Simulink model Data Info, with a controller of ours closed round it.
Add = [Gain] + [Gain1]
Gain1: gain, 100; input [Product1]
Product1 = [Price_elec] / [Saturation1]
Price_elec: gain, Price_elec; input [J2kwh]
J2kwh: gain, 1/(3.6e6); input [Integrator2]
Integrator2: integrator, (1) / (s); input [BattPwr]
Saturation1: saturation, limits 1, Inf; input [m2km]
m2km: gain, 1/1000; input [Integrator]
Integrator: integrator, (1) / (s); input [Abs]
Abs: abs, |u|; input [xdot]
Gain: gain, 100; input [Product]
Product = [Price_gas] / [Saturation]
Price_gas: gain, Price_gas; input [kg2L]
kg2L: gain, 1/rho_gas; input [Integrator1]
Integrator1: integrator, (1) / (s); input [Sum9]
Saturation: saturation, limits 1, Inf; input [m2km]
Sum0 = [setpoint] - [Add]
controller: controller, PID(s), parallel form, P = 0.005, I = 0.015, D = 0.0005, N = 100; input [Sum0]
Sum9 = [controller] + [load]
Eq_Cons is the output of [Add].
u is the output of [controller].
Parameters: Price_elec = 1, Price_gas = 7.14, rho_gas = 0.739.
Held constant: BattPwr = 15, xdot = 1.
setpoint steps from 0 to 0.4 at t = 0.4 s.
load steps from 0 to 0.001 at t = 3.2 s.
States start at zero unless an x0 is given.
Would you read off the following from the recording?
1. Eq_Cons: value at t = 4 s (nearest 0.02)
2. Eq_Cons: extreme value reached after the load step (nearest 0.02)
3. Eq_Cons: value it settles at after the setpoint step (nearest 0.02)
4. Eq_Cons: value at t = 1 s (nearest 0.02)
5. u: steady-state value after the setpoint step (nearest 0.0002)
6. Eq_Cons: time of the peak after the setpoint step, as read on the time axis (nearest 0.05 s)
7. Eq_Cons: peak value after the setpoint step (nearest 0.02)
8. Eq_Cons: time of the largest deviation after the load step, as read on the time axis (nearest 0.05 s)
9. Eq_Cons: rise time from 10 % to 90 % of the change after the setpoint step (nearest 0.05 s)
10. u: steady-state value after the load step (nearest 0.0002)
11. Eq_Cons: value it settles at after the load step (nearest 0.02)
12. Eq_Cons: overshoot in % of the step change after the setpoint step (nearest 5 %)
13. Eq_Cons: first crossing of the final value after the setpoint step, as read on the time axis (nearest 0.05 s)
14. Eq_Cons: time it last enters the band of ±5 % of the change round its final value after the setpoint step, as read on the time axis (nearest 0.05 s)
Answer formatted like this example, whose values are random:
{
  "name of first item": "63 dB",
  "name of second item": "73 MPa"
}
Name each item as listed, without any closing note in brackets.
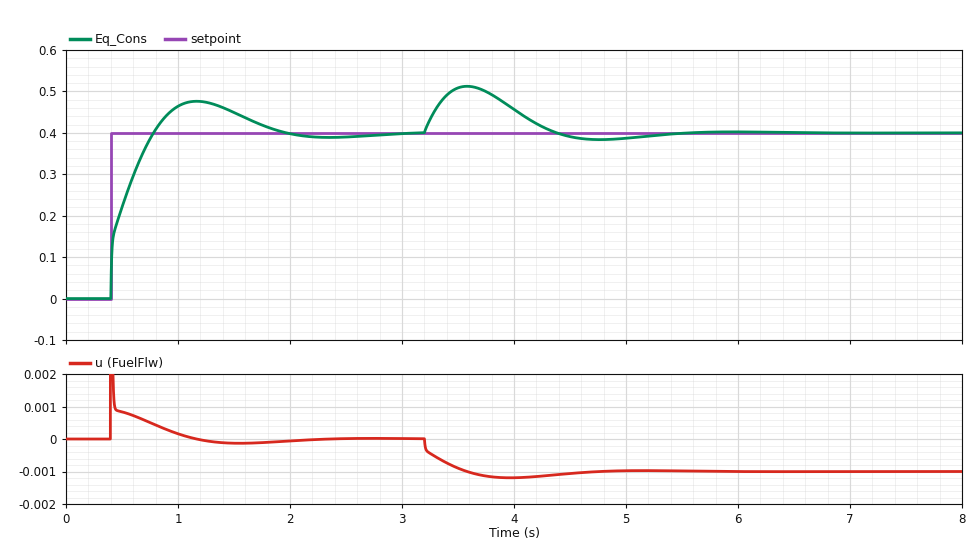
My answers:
{
  "Eq_Cons: value at t = 4 s": "0.46",
  "Eq_Cons: extreme value reached after the load step": "0.52",
  "Eq_Cons: value it settles at after the setpoint step": "0.40",
  "Eq_Cons: value at t = 1 s": "0.46",
  "u: steady-state value after the setpoint step": "0.0000",
  "Eq_Cons: time of the peak after the setpoint step, as read on the time axis": "1.15 s",
  "Eq_Cons: peak value after the setpoint step": "0.48",
  "Eq_Cons: time of the largest deviation after the load step, as read on the time axis": "3.60 s",
  "Eq_Cons: rise time from 10 % to 90 % of the change after the setpoint step": "0.30 s",
  "u: steady-state value after the load step": "-0.0010",
  "Eq_Cons: value it settles at after the load step": "0.40",
  "Eq_Cons: overshoot in % of the step change after the setpoint step": "20 %",
  "Eq_Cons: first crossing of the final value after the setpoint step, as read on the time axis": "0.80 s",
  "Eq_Cons: time it last enters the band of ±5 % of the change round its final value after the setpoint step, as read on the time axis": "1.75 s"
}
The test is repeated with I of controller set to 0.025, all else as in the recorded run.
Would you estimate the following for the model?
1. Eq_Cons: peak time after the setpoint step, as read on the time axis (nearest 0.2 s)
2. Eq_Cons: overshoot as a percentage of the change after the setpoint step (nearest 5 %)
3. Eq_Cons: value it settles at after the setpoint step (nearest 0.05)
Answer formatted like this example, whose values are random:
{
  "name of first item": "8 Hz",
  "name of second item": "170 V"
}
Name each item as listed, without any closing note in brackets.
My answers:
{
  "Eq_Cons: peak time after the setpoint step, as read on the time axis": "1.0 s",
  "Eq_Cons: overshoot as a percentage of the change after the setpoint step": "25 %",
  "Eq_Cons: value it settles at after the setpoint step": "0.40"
}
